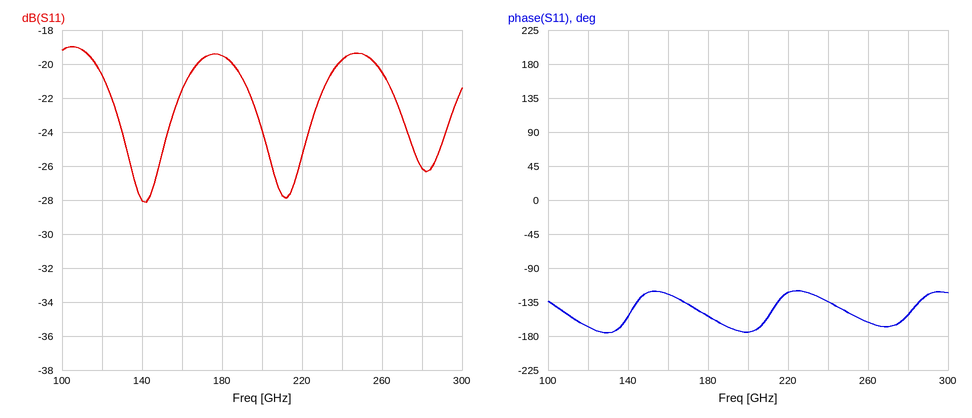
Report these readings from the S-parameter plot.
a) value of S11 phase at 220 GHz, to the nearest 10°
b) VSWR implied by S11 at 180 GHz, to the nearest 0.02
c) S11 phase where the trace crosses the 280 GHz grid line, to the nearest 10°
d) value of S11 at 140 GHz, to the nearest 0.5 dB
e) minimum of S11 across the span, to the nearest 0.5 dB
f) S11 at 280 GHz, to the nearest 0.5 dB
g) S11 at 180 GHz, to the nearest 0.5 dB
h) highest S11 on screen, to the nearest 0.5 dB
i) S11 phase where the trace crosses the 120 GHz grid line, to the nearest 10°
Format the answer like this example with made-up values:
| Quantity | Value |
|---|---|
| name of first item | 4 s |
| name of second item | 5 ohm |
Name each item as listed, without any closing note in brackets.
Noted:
| Quantity | Value |
|---|---|
| value of S11 phase at 220 GHz, to the nearest 10° | -120° |
| VSWR implied by S11 at 180 GHz, to the nearest 0.02 | 1.24 |
| S11 phase where the trace crosses the 280 GHz grid line, to the nearest 10° | -150° |
| value of S11 at 140 GHz, to the nearest 0.5 dB | -28.0 dB |
| minimum of S11 across the span, to the nearest 0.5 dB | -28.0 dB |
| S11 at 280 GHz, to the nearest 0.5 dB | -26.0 dB |
| S11 at 180 GHz, to the nearest 0.5 dB | -19.5 dB |
| highest S11 on screen, to the nearest 0.5 dB | -19.0 dB |
| S11 phase where the trace crosses the 120 GHz grid line, to the nearest 10° | -170° |
